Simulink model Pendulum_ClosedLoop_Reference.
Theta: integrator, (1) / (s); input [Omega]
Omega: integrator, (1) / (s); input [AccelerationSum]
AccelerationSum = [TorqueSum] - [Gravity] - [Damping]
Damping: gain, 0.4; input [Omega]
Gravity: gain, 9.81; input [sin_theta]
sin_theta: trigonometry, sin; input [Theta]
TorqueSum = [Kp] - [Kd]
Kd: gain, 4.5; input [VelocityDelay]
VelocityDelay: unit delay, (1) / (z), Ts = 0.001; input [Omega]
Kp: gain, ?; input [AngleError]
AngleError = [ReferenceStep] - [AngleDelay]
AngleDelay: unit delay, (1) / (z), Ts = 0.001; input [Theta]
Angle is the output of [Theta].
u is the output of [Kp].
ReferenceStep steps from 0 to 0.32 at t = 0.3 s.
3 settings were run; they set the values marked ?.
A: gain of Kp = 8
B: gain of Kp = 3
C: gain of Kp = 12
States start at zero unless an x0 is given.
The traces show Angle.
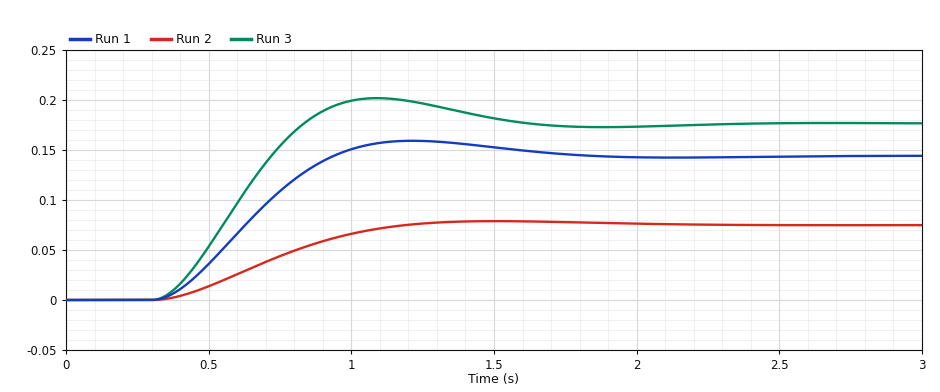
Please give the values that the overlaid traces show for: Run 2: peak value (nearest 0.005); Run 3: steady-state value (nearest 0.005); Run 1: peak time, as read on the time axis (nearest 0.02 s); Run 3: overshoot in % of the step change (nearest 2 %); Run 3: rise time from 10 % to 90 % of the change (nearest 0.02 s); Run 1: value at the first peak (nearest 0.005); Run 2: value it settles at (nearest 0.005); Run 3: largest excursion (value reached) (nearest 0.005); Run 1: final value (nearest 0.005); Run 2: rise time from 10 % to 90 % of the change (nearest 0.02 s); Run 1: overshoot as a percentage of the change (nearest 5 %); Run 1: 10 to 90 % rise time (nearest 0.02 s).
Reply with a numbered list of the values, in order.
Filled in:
1. 0.080
2. 0.175
3. 1.22 s
4. 14 %
5. 0.36 s
6. 0.160
7. 0.075
8. 0.200
9. 0.145
10. 0.58 s
11. 10 %
12. 0.42 s
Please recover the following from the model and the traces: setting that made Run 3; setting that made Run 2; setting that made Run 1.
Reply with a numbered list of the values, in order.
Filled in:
1. C
2. B
3. A
